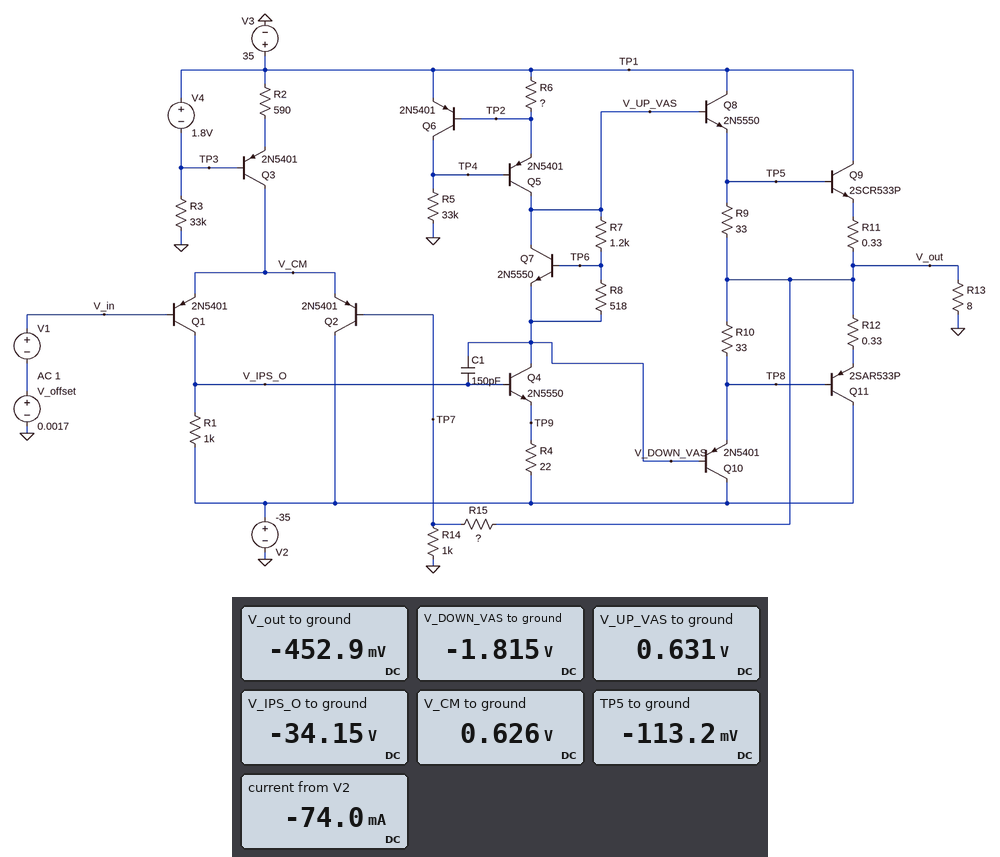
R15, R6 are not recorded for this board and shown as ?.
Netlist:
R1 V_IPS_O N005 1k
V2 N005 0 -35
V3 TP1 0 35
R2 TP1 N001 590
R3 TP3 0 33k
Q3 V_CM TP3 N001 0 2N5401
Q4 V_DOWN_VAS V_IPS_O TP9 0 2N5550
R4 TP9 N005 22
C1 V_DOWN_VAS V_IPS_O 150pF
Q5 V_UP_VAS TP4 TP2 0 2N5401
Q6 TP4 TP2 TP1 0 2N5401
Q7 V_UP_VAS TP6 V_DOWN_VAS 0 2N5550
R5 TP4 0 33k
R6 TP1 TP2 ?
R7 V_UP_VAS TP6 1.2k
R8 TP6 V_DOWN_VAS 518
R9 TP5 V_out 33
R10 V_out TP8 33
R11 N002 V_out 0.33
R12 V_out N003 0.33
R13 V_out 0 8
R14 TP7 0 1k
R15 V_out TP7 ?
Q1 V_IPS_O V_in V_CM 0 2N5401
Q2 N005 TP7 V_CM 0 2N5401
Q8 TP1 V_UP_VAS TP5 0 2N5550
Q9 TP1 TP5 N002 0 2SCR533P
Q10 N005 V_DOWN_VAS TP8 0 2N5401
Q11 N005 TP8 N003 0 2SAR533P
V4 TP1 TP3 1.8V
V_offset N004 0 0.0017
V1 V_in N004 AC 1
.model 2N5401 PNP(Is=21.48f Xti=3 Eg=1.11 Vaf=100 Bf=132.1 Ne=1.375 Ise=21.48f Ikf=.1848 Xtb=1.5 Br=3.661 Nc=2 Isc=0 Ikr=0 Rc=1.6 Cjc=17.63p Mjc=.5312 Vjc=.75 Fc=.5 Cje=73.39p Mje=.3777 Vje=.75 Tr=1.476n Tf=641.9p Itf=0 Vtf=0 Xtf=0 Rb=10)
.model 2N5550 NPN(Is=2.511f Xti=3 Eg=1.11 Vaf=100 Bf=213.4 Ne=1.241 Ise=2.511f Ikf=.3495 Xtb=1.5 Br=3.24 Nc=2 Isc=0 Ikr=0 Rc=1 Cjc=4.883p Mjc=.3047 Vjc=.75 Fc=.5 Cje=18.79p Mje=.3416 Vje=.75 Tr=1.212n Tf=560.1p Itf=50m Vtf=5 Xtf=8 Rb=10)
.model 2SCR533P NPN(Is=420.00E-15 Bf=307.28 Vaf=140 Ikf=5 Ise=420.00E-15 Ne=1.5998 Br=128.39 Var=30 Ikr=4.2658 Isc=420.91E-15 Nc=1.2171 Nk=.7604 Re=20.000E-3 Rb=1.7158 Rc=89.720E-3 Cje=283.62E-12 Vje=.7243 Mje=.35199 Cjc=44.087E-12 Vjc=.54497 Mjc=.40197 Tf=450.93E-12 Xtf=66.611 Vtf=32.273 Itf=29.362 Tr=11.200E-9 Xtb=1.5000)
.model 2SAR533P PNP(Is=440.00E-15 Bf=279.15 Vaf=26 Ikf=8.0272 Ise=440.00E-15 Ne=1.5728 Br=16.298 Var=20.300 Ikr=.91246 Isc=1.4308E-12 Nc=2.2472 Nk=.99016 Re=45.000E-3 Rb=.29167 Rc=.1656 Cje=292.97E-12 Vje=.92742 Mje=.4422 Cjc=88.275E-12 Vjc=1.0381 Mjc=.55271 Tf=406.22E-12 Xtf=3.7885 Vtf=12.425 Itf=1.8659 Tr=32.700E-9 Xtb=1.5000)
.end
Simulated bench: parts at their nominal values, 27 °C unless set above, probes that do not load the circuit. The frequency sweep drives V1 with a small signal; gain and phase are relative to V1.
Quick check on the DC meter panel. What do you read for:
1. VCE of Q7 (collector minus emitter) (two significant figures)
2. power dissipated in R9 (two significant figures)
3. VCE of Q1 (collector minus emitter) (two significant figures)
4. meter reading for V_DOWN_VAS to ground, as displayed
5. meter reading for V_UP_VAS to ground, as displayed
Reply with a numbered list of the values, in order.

1. 2.4 V
2. 3.5 mW
3. -35 V
4. -1.815 V
5. 0.631 V
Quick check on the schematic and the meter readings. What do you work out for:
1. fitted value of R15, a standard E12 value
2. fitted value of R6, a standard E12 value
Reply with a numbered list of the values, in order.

1. 47 kΩ
2. 120 Ω
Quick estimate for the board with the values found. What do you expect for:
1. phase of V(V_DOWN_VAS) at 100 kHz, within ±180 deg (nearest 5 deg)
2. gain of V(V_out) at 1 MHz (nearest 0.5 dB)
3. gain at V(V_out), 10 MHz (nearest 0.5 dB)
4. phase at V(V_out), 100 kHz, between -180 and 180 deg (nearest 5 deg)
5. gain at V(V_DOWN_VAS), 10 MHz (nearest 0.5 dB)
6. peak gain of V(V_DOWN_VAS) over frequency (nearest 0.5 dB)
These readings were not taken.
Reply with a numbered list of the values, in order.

1. -20 deg
2. 23.5 dB
3. -8.0 dB
4. -20 deg
5. -7.0 dB
6. 34.5 dB
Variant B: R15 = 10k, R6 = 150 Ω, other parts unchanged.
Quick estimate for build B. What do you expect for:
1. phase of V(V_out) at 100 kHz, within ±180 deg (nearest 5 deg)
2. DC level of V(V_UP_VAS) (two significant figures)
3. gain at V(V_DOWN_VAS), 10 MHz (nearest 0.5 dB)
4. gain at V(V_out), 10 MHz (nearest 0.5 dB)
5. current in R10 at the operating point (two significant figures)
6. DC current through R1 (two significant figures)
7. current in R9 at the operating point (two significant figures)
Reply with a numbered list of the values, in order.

1. -5 deg
2. 990 mV
3. -6.0 dB
4. -8.5 dB
5. 18 mA
6. 820 µA
7. 11 mA
